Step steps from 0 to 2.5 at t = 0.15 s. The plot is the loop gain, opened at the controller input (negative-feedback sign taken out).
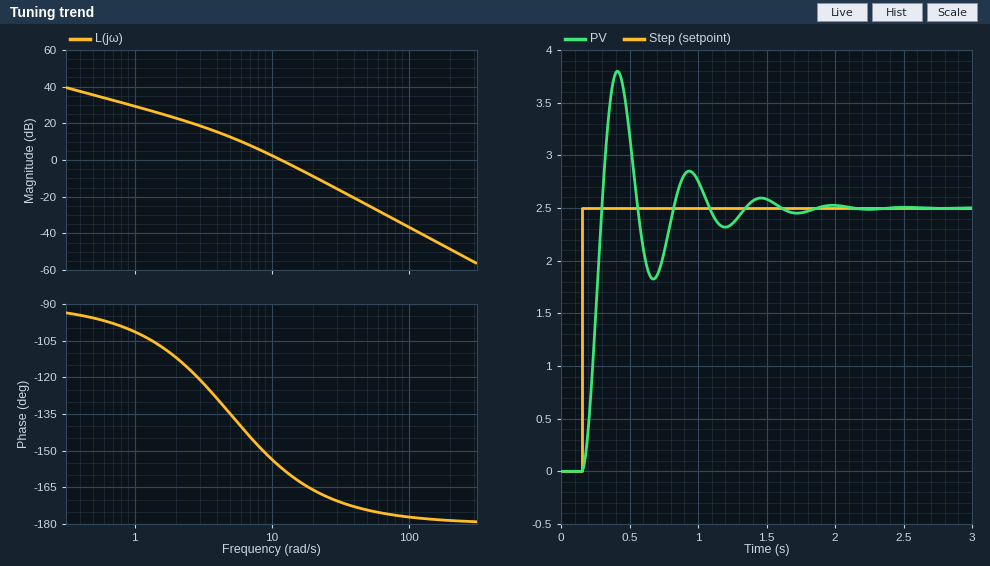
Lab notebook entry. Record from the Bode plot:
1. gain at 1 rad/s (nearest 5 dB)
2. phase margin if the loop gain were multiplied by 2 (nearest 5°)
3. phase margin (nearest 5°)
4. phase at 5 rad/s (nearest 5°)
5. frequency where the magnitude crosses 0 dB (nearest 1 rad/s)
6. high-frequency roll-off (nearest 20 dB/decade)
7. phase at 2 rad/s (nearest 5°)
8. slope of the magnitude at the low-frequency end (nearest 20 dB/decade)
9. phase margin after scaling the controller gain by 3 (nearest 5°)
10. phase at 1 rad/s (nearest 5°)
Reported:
30 dB
15°
25°
-135°
12 rad/s
-40 dB/decade
-110°
-20 dB/decade
15°
-100°
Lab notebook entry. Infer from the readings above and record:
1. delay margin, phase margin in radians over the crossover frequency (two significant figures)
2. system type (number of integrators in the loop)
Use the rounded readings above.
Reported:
0.036 s
1
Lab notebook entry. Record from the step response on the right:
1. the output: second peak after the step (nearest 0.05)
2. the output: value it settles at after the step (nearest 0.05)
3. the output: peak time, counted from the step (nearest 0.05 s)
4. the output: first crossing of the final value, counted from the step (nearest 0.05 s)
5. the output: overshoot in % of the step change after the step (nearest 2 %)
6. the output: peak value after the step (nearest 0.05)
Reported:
2.85
2.50
0.25 s
0.15 s
52 %
3.80
